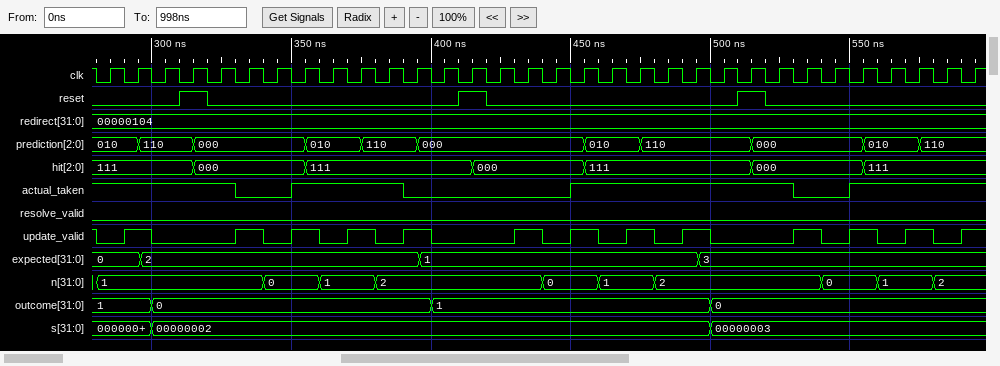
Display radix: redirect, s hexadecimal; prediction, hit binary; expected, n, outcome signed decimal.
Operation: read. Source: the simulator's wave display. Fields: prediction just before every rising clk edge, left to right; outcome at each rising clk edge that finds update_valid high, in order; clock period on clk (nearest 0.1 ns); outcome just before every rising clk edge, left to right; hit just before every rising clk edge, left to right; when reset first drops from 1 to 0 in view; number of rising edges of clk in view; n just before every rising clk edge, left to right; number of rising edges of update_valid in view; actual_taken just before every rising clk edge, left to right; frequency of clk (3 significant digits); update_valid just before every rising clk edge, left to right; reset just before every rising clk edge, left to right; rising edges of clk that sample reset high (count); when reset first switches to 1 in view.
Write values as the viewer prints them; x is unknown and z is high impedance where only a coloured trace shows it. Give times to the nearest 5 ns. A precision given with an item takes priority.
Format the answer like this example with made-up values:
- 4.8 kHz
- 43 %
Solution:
- 010, 010, 110, 110, 000, 000, 000, 000, 010, 010, 110, 110, 000, 000, 000, 000, 000, 000, 010, 010, 110, 110, 110, 110, 000, 000, 000, 000, 010, 010, 110, 110
- 1, 0, 0, 0, 0, 1, 1, 1, 1, 0, 0, 0, 0
- 10 ns
- 1, 1, 0, 0, 0, 0, 0, 0, 0, 0, 0, 0, 1, 1, 1, 1, 1, 1, 1, 1, 1, 1, 0, 0, 0, 0, 0, 0, 0, 0, 0, 0
- 111, 111, 111, 111, 000, 000, 000, 000, 111, 111, 111, 111, 111, 111, 000, 000, 000, 000, 111, 111, 111, 111, 111, 111, 000, 000, 000, 000, 111, 111, 111, 111
- 320 ns
- 32
- 1, 1, 1, 1, 1, 1, 0, 0, 1, 1, 2, 2, 2, 2, 2, 2, 0, 0, 1, 1, 2, 2, 2, 2, 2, 2, 0, 0, 1, 1, 2, 2
- 13
- 1 1 1 1 1 0 0 1 1 1 1 0 0 0 0 0 0 1 1 1 1 1 1 1 1 0 0 1 1 1 1 1
- 100 MHz
- 0 1 0 0 0 1 0 1 0 1 0 1 0 0 0 1 0 1 0 1 0 1 0 0 0 1 0 1 0 1 0 1
- 0 0 0 1 0 0 0 0 0 0 0 0 0 1 0 0 0 0 0 0 0 0 0 1 0 0 0 0 0 0 0 0
- 3
- 310 ns
